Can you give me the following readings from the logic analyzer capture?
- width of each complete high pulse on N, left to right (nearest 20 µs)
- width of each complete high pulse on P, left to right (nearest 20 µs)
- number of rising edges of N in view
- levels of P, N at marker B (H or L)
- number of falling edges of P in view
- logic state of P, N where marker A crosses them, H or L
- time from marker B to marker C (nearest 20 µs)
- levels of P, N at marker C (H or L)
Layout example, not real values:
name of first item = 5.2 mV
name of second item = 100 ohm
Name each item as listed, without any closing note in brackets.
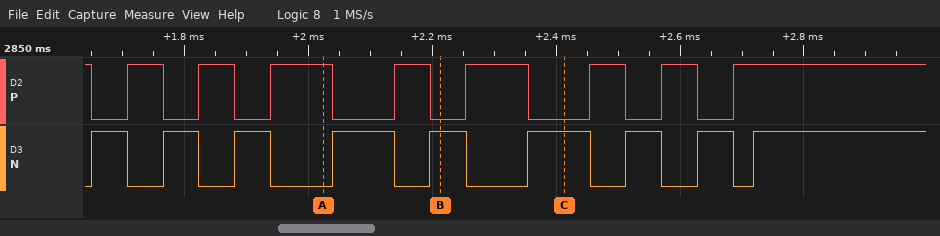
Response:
width of each complete high pulse on N, left to right = 60 µs, 60 µs, 60 µs, 100 µs, 60 µs, 100 µs, 60 µs, 60 µs
width of each complete high pulse on P, left to right = 60 µs, 60 µs, 100 µs, 60 µs, 100 µs, 60 µs, 60 µs
number of rising edges of N in view = 9
levels of P, N at marker B = P=L, N=H
number of falling edges of P in view = 8
logic state of P, N where marker A crosses them, H or L = P=H, N=L
time from marker B to marker C = 200 µs
levels of P, N at marker C = P=L, N=H
